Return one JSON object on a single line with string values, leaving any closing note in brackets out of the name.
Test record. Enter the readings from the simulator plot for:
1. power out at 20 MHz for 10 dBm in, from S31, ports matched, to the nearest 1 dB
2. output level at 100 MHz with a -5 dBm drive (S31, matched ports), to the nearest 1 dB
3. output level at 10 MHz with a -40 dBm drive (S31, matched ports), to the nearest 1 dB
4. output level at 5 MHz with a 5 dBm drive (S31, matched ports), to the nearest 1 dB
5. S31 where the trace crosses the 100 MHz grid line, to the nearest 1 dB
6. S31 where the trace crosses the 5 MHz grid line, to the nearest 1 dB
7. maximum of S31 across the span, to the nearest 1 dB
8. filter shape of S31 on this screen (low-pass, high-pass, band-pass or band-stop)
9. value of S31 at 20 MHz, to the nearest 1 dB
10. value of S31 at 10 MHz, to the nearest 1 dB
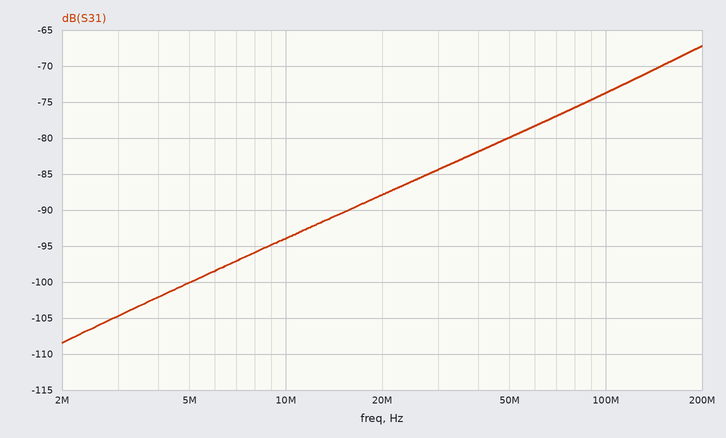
{"power out at 20 MHz for 10 dBm in, from S31, ports matched, to the nearest 1 dB": "-78 dBm", "output level at 100 MHz with a -5 dBm drive (S31, matched ports), to the nearest 1 dB": "-79 dBm", "output level at 10 MHz with a -40 dBm drive (S31, matched ports), to the nearest 1 dB": "-134 dBm", "output level at 5 MHz with a 5 dBm drive (S31, matched ports), to the nearest 1 dB": "-95 dBm", "S31 where the trace crosses the 100 MHz grid line, to the nearest 1 dB": "-74 dB", "S31 where the trace crosses the 5 MHz grid line, to the nearest 1 dB": "-100 dB", "maximum of S31 across the span, to the nearest 1 dB": "-67 dB", "filter shape of S31 on this screen": "high-pass", "value of S31 at 20 MHz, to the nearest 1 dB": "-88 dB", "value of S31 at 10 MHz, to the nearest 1 dB": "-94 dB"}
